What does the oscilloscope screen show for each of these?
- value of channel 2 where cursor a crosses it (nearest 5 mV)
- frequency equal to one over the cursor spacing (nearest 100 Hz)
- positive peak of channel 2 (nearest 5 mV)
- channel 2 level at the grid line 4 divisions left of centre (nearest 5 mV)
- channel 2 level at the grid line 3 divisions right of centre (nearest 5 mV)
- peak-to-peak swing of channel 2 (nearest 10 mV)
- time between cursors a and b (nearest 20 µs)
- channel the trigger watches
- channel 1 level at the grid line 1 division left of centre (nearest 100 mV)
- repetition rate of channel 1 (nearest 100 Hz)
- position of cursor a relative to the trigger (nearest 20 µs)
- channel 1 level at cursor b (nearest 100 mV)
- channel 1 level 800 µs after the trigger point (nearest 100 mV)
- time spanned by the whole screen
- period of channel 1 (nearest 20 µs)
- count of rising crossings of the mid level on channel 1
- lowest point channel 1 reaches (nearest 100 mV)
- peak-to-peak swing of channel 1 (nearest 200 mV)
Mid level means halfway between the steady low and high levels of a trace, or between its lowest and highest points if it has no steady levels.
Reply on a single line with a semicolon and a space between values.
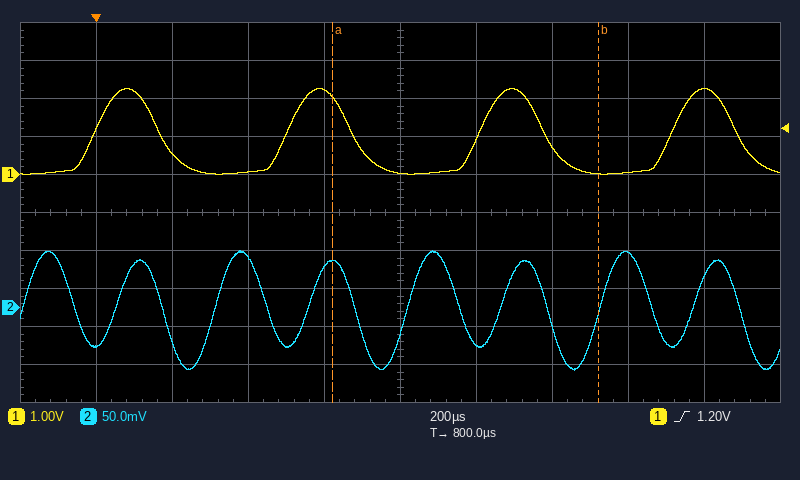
60 mV; 1.4 kHz; 75 mV; -50 mV; 70 mV; 160 mV; 700 µs; channel 1; 2.2 V; 2.0 kHz; +620 µs; 0.0 V; 0.0 V; 2 ms; 500 µs; 4; 0.0 V; 2.2 V
